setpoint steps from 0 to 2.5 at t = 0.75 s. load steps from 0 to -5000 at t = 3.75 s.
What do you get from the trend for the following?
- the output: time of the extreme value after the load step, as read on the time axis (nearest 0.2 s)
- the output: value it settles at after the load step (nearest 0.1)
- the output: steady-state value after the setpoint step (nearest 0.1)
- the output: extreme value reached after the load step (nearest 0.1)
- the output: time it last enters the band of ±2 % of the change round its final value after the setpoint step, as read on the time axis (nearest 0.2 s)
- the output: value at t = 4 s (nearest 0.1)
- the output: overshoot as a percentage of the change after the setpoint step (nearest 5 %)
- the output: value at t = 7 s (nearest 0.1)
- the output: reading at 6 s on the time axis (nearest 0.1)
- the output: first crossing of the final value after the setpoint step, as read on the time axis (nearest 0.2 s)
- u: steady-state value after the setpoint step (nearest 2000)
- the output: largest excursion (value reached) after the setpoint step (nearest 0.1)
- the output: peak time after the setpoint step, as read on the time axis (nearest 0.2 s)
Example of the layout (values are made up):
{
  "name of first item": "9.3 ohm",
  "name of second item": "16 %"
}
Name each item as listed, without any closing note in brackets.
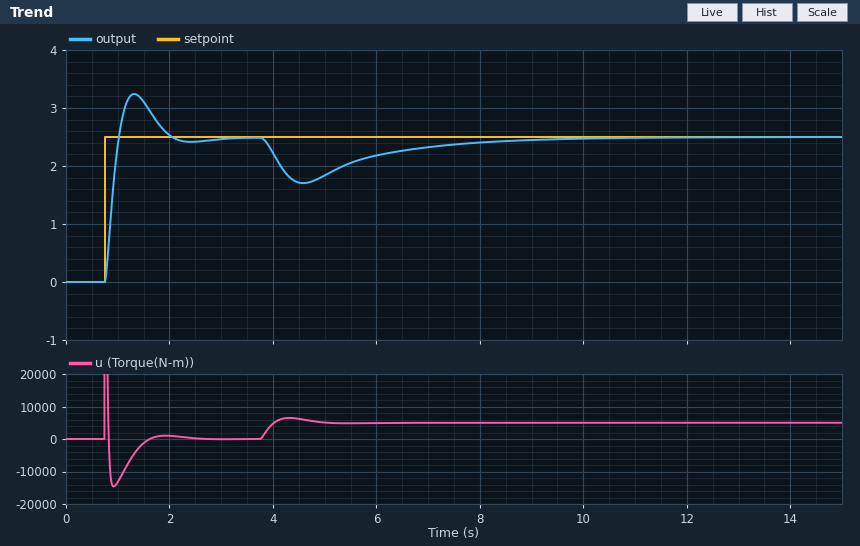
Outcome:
{
  "the output: time of the extreme value after the load step, as read on the time axis": "4.6 s",
  "the output: value it settles at after the load step": "2.5",
  "the output: steady-state value after the setpoint step": "2.5",
  "the output: extreme value reached after the load step": "1.7",
  "the output: time it last enters the band of ±2 % of the change round its final value after the setpoint step, as read on the time axis": "2.8 s",
  "the output: value at t = 4 s": "2.2",
  "the output: overshoot as a percentage of the change after the setpoint step": "30 %",
  "the output: value at t = 7 s": "2.3",
  "the output: reading at 6 s on the time axis": "2.2",
  "the output: first crossing of the final value after the setpoint step, as read on the time axis": "1.0 s",
  "u: steady-state value after the setpoint step": "0",
  "the output: largest excursion (value reached) after the setpoint step": "3.2",
  "the output: peak time after the setpoint step, as read on the time axis": "1.4 s"
}
